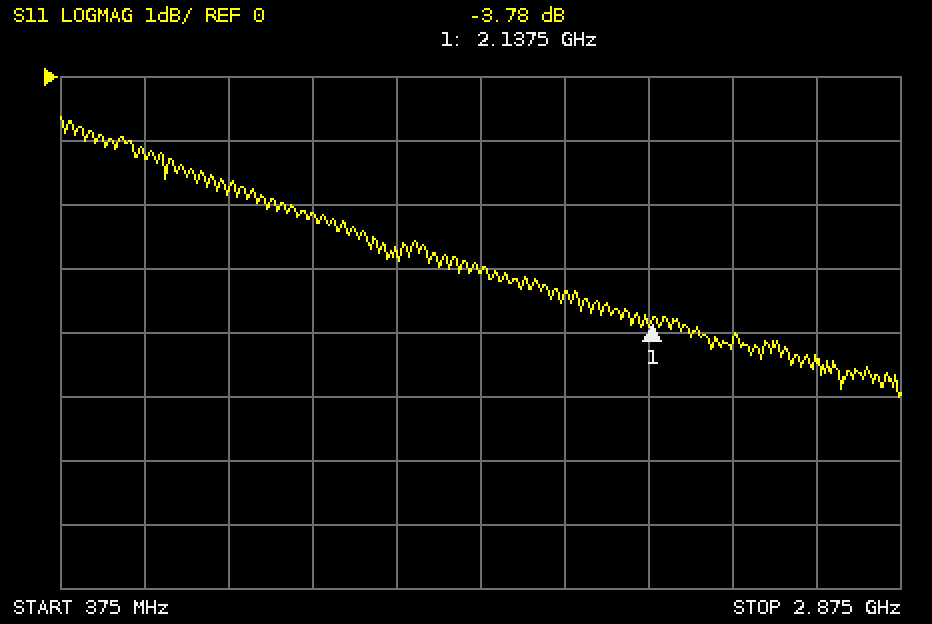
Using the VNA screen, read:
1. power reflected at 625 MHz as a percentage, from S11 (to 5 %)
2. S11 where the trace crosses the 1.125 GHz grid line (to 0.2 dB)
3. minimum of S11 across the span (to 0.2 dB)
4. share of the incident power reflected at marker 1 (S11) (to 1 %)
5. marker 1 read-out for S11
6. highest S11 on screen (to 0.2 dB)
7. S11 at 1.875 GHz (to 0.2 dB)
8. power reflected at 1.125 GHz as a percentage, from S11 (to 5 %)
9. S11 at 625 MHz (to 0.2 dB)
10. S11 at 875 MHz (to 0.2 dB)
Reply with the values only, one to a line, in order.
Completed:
75 %
-2.2 dB
-5.0 dB
42 %
-3.78 dB
-0.6 dB
-3.4 dB
60 %
-1.2 dB
-1.8 dB
